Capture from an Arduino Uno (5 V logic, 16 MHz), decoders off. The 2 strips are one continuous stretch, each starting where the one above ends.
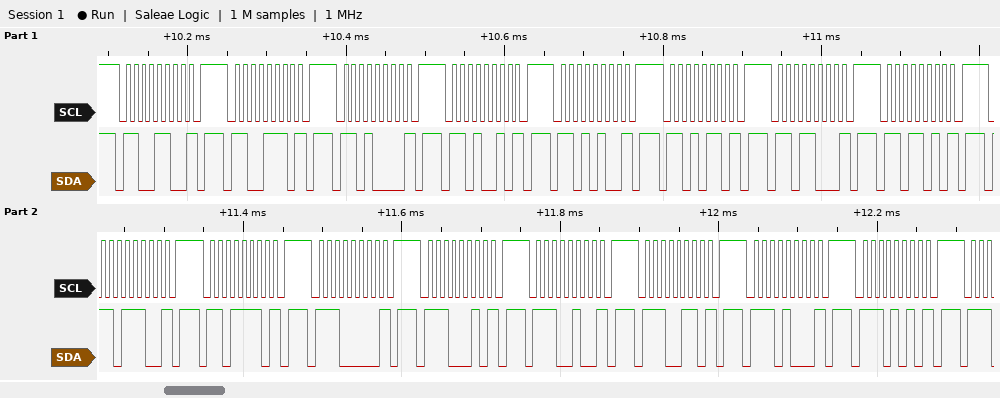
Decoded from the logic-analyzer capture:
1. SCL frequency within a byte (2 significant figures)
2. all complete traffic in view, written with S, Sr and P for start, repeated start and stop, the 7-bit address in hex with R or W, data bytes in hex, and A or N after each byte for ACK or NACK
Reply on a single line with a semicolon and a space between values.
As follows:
100 kHz; S 66W N P S 67W N P S 68W N P S 69W N P S 6AW N P S 6BW N P S 6CW N P S 6DW N P S 6EW N P S 6FW N P S 70W N P S 71W N P S 72W N P S 73W N P S 74W N P S 75W N P
